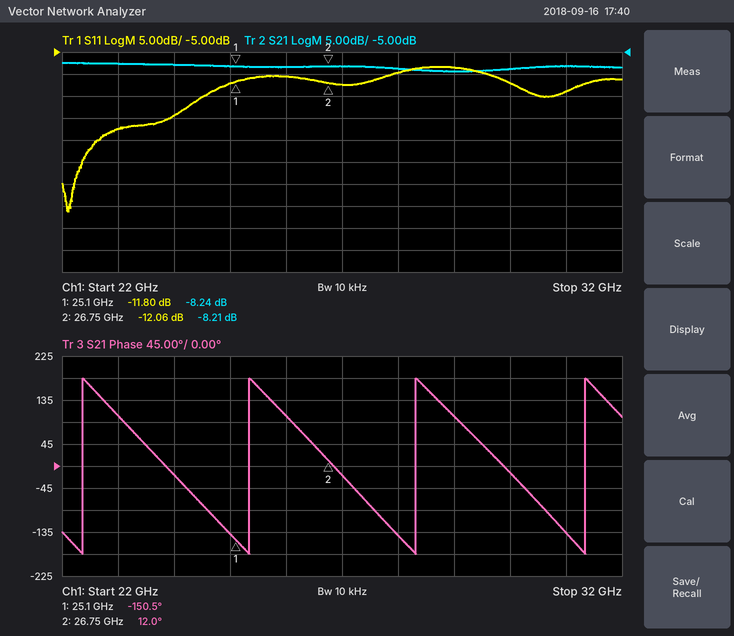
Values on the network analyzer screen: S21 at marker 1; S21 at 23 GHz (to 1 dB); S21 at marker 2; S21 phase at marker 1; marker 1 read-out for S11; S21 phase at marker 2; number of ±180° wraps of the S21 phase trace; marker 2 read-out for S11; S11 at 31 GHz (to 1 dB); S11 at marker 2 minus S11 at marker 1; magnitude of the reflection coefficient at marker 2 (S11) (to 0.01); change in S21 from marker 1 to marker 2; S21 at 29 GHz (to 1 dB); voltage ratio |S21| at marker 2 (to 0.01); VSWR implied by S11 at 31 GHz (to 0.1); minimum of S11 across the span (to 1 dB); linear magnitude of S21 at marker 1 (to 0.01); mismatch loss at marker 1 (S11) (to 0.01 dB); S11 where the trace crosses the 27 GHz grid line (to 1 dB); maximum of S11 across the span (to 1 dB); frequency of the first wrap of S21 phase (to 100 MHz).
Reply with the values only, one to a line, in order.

-8.24 dB
-8 dB
-8.21 dB
-150.5°
-11.80 dB
12.0°
4
-12.06 dB
-14 dB
-0.26 dB
0.25
0.03 dB
-9 dB
0.39
1.5
-41 dB
0.39
0.30 dB
-12 dB
-8 dB
22.4 GHz
